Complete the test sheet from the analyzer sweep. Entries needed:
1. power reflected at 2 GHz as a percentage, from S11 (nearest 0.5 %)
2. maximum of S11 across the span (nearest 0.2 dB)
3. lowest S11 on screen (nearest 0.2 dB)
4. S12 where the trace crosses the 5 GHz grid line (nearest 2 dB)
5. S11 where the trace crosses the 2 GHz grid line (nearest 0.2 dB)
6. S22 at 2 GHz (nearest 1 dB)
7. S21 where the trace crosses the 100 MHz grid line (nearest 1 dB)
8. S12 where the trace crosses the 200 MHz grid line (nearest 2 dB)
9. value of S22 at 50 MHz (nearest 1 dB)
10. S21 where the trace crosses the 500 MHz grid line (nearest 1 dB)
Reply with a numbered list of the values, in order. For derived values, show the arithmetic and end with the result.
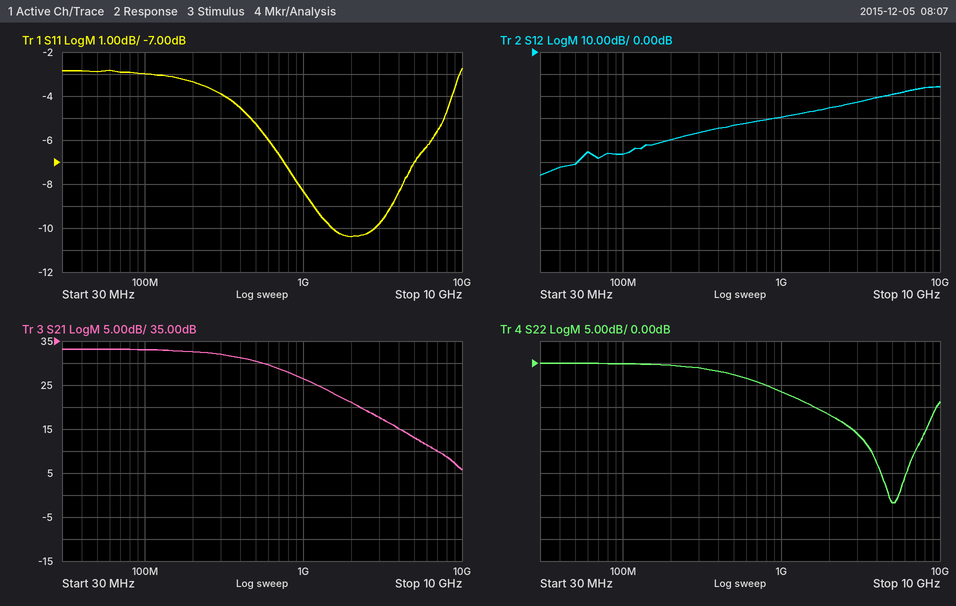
1. 10^(-10.4/10) ≈ 9.12 %, so 9.0 % to the nearest 0.5 %
2. -2.8 dB
3. -10.4 dB
4. -20 dB
5. -10.4 dB
6. -12 dB
7. 33 dB
8. -40 dB
9. 0 dB
10. 30 dB
